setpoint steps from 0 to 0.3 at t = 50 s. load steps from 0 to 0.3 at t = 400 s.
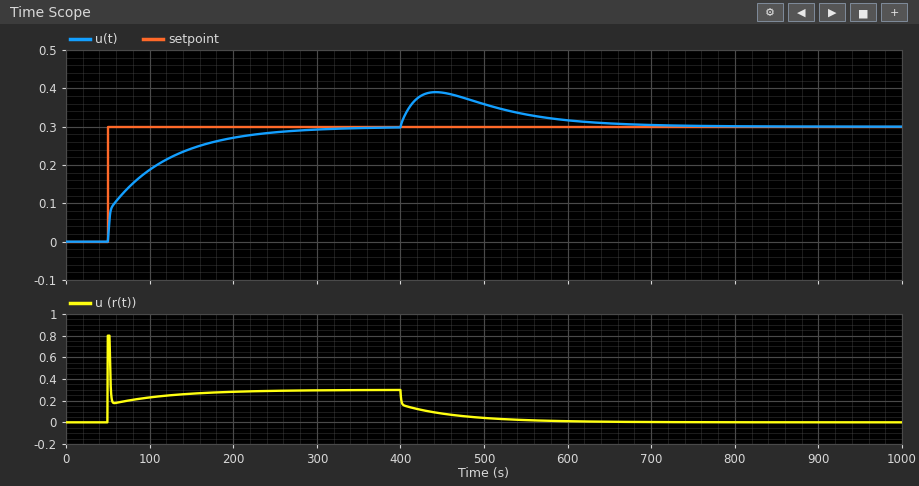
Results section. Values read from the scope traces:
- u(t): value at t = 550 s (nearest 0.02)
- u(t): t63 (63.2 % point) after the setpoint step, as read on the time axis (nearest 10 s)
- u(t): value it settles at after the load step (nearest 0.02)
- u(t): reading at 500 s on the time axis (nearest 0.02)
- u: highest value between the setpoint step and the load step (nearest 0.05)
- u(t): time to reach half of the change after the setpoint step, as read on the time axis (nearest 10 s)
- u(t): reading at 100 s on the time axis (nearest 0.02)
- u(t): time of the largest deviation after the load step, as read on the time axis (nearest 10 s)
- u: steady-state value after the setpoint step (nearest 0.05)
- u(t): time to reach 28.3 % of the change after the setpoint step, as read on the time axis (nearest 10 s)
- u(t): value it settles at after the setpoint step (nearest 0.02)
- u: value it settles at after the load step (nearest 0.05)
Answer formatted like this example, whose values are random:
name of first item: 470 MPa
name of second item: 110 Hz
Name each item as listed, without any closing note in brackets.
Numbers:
u(t): value at t = 550 s: 0.34
u(t): t63 (63.2 % point) after the setpoint step, as read on the time axis: 100 s
u(t): value it settles at after the load step: 0.30
u(t): reading at 500 s on the time axis: 0.36
u: highest value between the setpoint step and the load step: 0.80
u(t): time to reach half of the change after the setpoint step, as read on the time axis: 80 s
u(t): reading at 100 s on the time axis: 0.18
u(t): time of the largest deviation after the load step, as read on the time axis: 440 s
u: steady-state value after the setpoint step: 0.30
u(t): time to reach 28.3 % of the change after the setpoint step, as read on the time axis: 50 s
u(t): value it settles at after the setpoint step: 0.30
u: value it settles at after the load step: 0.00
